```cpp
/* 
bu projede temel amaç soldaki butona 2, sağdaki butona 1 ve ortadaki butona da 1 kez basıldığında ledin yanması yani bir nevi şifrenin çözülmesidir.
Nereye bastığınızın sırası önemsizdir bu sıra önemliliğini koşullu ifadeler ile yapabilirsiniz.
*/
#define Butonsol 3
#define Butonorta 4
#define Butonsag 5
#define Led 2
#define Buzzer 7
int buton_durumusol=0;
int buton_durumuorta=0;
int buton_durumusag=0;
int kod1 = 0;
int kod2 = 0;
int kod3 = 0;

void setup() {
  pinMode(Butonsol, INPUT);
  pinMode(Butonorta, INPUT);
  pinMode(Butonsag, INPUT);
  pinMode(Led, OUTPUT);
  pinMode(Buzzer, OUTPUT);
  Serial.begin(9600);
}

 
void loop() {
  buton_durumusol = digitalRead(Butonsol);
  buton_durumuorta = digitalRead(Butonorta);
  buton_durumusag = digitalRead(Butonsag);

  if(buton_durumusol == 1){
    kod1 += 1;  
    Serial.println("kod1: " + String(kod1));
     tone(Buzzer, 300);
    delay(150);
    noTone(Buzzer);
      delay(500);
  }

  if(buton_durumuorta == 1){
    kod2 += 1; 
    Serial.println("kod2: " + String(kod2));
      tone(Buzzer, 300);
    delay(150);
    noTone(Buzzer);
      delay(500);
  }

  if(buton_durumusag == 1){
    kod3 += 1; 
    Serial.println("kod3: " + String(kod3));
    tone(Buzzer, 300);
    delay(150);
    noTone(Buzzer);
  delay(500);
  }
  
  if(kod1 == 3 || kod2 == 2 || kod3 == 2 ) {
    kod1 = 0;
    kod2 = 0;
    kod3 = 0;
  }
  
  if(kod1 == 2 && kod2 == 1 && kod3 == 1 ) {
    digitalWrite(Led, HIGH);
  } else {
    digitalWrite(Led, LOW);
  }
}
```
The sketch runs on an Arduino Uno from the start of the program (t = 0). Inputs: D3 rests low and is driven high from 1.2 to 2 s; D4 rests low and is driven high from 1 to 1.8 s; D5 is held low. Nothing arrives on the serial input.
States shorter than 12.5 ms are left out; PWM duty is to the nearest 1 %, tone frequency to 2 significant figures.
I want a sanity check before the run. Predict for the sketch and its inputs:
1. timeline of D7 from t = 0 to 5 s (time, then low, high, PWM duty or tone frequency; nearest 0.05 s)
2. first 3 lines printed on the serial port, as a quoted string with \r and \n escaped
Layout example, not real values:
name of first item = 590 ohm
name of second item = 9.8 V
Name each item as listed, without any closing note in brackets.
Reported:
timeline of D7 from t = 0 to 5 s = 0 s low; 1 s tone 300 Hz; 1.15 s low; 1.65 s tone 300 Hz; 1.8 s low; 2.3 s tone 300 Hz; 2.45 s low
first 3 lines printed on the serial port, as a quoted string with \r and \n escaped = "kod2: 1\r\nkod1: 1\r\nkod2: 2\r\n"
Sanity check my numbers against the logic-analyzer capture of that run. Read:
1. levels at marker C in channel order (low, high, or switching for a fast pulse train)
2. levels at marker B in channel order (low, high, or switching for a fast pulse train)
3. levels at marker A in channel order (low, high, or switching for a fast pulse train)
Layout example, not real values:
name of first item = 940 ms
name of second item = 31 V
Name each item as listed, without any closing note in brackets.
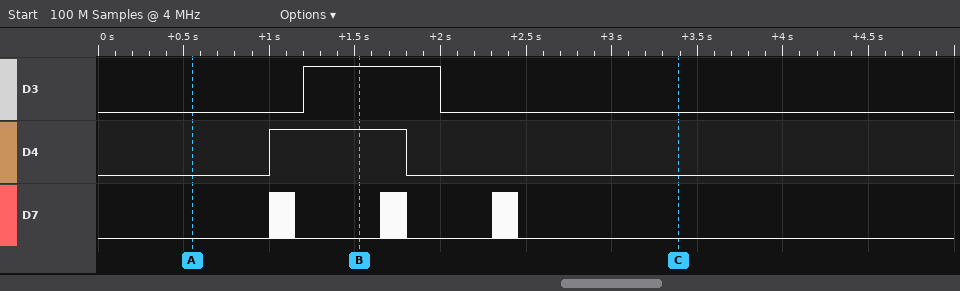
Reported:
levels at marker C in channel order = D3 low, D4 low, D7 low
levels at marker B in channel order = D3 high, D4 high, D7 low
levels at marker A in channel order = D3 low, D4 low, D7 low
